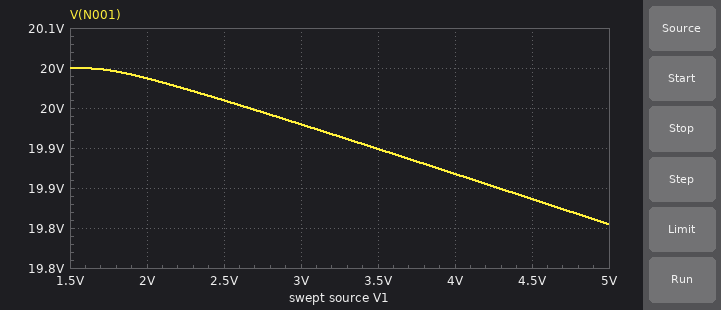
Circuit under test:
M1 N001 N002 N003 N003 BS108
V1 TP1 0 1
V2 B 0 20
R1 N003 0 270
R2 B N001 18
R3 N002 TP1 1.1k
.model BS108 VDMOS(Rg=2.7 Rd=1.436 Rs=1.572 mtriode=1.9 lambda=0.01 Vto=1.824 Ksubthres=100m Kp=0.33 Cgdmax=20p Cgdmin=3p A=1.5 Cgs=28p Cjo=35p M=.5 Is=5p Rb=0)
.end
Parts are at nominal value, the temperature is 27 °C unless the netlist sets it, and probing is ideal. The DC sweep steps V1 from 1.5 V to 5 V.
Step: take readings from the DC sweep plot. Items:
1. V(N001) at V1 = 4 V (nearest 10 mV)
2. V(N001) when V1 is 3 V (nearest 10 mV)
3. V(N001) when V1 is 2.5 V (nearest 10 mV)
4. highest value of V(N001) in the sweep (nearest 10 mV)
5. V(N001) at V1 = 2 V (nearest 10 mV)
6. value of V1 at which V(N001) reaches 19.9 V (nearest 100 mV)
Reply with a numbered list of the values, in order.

1. 19.87 V
2. 19.93 V
3. 19.96 V
4. 20.00 V
5. 19.99 V
6. 3.5 V
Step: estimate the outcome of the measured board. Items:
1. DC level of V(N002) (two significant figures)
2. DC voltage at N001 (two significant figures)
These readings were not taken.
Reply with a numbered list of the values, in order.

1. 1.0 V
2. 20 V
